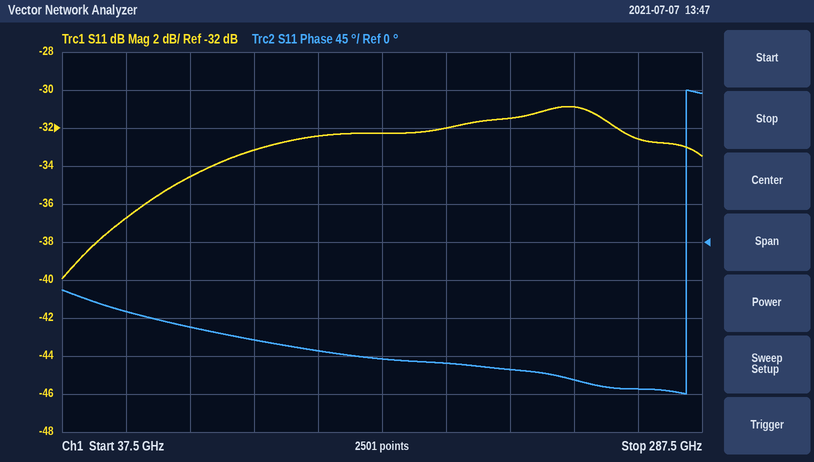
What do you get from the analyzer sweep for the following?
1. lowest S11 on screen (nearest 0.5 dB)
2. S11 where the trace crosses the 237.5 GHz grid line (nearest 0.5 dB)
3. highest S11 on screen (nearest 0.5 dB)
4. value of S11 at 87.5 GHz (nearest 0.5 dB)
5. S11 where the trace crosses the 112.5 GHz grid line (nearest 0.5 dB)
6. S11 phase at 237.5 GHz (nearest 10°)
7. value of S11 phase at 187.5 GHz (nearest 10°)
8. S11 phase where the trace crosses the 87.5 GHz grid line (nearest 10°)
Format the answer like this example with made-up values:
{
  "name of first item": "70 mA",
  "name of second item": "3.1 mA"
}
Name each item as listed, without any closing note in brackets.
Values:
{
  "lowest S11 on screen": "-40.0 dB",
  "S11 where the trace crosses the 237.5 GHz grid line": "-31.0 dB",
  "highest S11 on screen": "-31.0 dB",
  "value of S11 at 87.5 GHz": "-34.5 dB",
  "S11 where the trace crosses the 112.5 GHz grid line": "-33.0 dB",
  "S11 phase at 237.5 GHz": "-160°",
  "value of S11 phase at 187.5 GHz": "-140°",
  "S11 phase where the trace crosses the 87.5 GHz grid line": "-100°"
}
